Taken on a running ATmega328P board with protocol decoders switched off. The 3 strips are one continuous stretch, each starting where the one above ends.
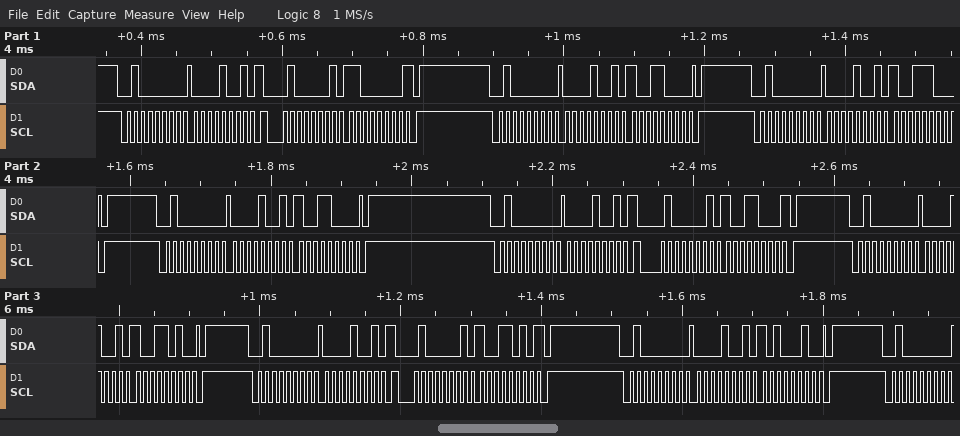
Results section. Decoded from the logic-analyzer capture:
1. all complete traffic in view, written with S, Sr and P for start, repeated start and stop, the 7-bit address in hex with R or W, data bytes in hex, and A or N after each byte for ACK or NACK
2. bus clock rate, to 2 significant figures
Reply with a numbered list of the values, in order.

1. S 20W A 09 A Sr 20R A C0 N P S 20W A 09 A 98 A P S 20W A 09 A 9C A P S 20W A 09 A 98 A P S 20W A 09 A Sr 20R A 98 N P S 20W A 09 A 9A A P S 20W A 09 A Sr 20R A 9A N P S 20W A 09 A A2 A P S 20W A
2. 100 kHz
